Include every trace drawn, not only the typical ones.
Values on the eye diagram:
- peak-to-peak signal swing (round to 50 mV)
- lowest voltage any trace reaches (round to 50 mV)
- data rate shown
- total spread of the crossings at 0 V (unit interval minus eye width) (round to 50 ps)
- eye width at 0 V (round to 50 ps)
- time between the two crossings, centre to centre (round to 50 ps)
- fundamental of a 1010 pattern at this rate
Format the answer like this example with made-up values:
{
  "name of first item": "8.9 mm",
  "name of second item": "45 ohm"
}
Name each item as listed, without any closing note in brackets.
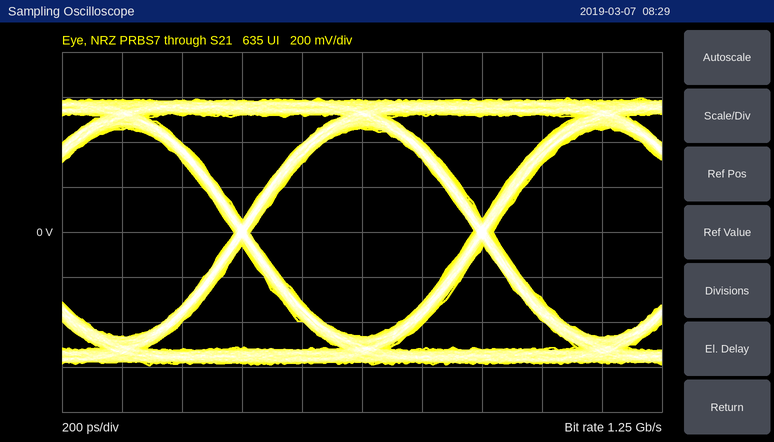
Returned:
{
  "peak-to-peak signal swing": "1.20 V",
  "lowest voltage any trace reaches": "-600 mV",
  "data rate shown": "1.25 Gb/s",
  "total spread of the crossings at 0 V (unit interval minus eye width)": "50 ps",
  "eye width at 0 V": "750 ps",
  "time between the two crossings, centre to centre": "800 ps",
  "fundamental of a 1010 pattern at this rate": "625 MHz"
}
